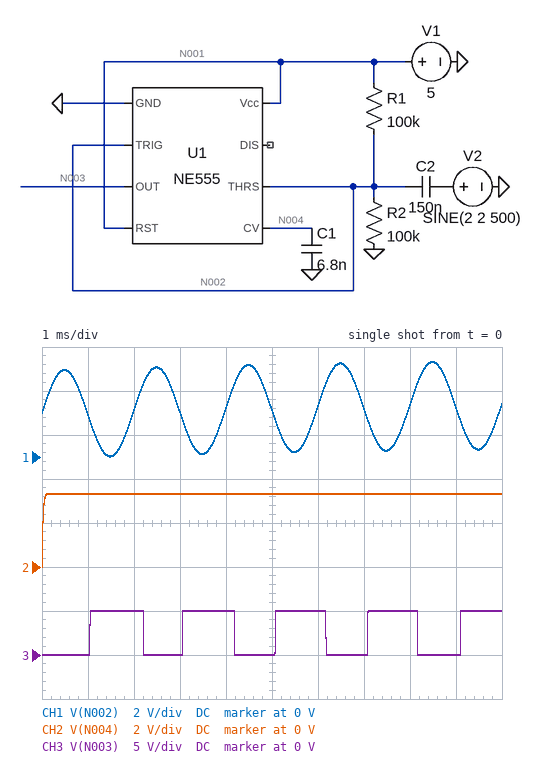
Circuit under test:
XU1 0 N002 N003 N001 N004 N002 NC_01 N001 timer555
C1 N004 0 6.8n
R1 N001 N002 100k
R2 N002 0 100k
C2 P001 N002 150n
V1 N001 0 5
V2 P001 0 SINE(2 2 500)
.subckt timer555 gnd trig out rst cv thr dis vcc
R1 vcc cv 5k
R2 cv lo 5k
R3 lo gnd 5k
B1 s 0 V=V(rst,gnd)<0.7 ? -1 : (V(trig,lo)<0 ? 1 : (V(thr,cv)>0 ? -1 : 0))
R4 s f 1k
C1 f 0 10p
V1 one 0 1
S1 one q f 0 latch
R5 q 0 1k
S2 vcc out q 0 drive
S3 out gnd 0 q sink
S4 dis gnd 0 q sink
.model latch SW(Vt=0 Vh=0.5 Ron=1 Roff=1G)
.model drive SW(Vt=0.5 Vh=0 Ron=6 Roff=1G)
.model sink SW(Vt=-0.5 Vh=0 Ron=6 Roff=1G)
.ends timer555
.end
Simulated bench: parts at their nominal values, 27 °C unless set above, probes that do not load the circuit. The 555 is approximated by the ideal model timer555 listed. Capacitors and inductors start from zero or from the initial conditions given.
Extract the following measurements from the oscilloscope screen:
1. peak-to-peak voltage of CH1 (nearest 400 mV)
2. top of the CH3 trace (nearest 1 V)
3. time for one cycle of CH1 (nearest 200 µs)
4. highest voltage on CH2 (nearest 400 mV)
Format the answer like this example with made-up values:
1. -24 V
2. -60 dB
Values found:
1. 4.4 V
2. 5 V
3. 2.0 ms
4. 3.2 V
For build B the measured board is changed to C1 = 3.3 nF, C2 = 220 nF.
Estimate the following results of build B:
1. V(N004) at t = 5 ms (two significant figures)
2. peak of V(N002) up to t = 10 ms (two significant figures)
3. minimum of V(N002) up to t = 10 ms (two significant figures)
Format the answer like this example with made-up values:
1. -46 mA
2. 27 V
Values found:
1. 3.3 V
2. 4.2 V
3. 14 mV
